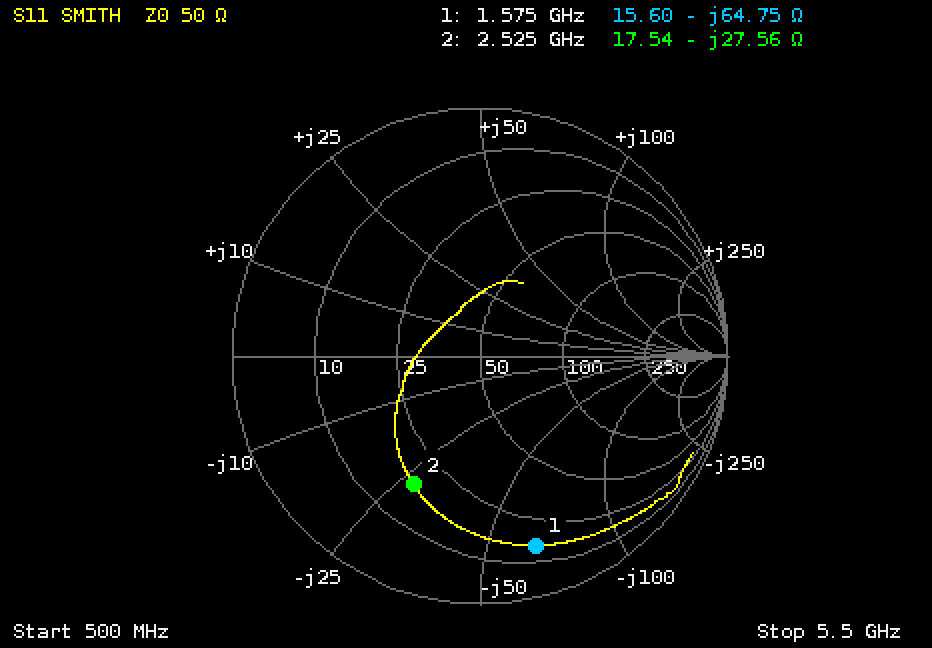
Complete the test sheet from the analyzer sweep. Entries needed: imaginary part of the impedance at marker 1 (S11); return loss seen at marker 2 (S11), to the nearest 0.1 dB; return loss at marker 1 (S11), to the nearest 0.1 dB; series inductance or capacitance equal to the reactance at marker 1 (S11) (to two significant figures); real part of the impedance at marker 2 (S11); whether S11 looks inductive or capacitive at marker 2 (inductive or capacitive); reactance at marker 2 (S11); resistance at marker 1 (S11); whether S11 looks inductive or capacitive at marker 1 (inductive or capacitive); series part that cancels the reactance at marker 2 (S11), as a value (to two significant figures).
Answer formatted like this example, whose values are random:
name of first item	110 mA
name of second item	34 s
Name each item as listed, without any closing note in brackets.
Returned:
imaginary part of the impedance at marker 1	-64.75 Ω
return loss seen at marker 2 (S11), to the nearest 0.1 dB	4.7 dB
return loss at marker 1 (S11), to the nearest 0.1 dB	2.0 dB
series inductance or capacitance equal to the reactance at marker 1 (S11)	1.6 pF
real part of the impedance at marker 2	17.54 Ω
whether S11 looks inductive or capacitive at marker 2	capacitive
reactance at marker 2	-27.56 Ω
resistance at marker 1	15.60 Ω
whether S11 looks inductive or capacitive at marker 1	capacitive
series part that cancels the reactance at marker 2 (S11), as a value	1.7 nH
